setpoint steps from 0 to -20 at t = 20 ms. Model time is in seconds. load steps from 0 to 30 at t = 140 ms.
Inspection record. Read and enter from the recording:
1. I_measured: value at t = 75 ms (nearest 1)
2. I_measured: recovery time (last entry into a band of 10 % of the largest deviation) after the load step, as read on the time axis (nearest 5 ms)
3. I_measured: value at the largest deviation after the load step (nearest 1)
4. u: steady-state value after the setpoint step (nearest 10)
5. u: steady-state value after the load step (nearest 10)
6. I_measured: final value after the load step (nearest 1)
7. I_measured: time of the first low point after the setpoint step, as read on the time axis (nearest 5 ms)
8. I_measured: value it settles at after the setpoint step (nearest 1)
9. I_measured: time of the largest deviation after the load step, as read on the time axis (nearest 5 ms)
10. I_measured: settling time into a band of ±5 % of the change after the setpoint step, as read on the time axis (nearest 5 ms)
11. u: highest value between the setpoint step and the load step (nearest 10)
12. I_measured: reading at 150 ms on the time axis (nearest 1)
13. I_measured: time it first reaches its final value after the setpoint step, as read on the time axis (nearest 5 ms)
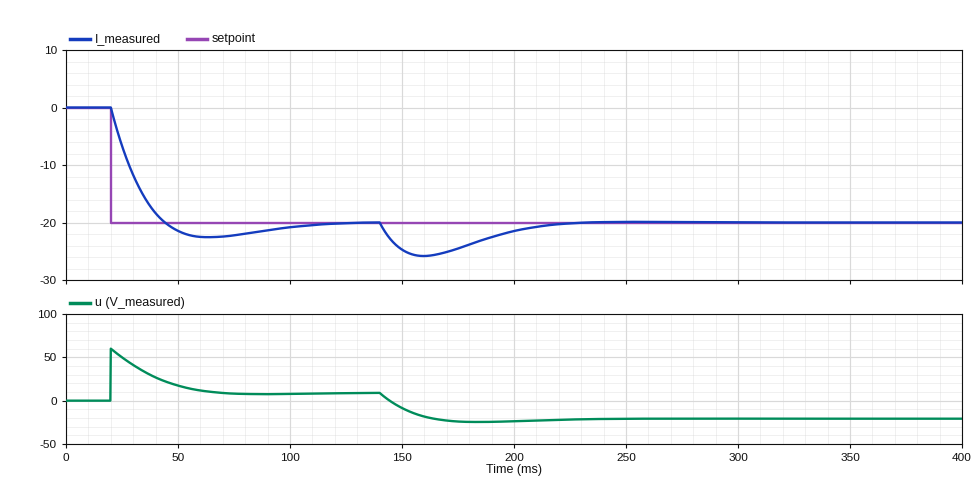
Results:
-22
215 ms
-26
10
-20
-20
65 ms
-20
160 ms
95 ms
60
-25
45 ms
